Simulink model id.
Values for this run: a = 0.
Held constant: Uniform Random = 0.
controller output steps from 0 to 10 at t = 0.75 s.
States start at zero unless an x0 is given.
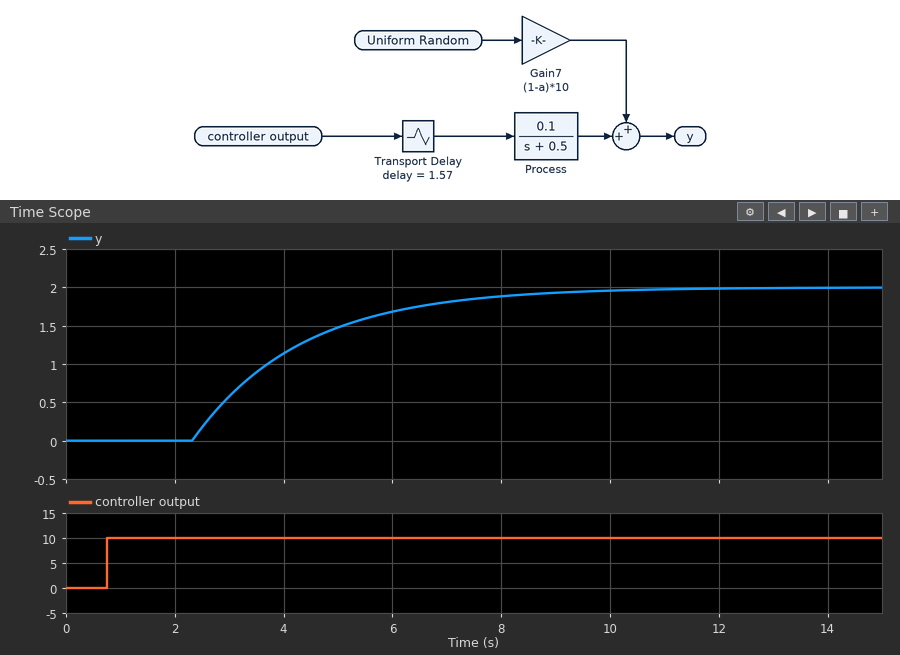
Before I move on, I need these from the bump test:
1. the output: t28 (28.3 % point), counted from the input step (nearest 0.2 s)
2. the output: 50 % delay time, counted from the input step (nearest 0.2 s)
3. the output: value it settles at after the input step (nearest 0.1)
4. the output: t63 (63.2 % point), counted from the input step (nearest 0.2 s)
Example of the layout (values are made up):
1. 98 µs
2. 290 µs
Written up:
1. 2.2 s
2. 3.0 s
3. 2.0
4. 3.6 s
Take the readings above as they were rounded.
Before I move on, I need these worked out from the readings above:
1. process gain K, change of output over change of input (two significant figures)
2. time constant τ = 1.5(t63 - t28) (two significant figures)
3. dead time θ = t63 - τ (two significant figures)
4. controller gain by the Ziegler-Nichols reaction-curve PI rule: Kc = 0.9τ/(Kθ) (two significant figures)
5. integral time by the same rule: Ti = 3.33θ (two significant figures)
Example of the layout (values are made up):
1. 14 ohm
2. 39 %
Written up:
1. 0.20
2. 2.1 s
3. 1.5 s
4. 6.3
5. 5.0 s
